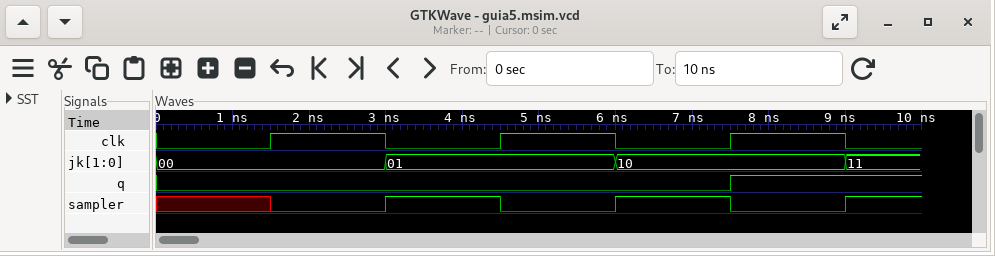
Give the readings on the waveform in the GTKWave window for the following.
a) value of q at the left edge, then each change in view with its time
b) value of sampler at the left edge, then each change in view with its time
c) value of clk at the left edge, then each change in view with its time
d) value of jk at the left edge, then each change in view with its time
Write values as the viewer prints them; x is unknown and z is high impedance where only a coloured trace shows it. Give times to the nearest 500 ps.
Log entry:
0, 1 at 7500 ps
x, 0 at 1500 ps, 1 at 3000 ps, 0 at 4500 ps, 1 at 6000 ps, 0 at 7500 ps, 1 at 9000 ps
0, 1 at 1500 ps, 0 at 3000 ps, 1 at 4500 ps, 0 at 6000 ps, 1 at 7500 ps, 0 at 9000 ps
00, 01 at 3000 ps, 10 at 6000 ps, 11 at 9000 ps
